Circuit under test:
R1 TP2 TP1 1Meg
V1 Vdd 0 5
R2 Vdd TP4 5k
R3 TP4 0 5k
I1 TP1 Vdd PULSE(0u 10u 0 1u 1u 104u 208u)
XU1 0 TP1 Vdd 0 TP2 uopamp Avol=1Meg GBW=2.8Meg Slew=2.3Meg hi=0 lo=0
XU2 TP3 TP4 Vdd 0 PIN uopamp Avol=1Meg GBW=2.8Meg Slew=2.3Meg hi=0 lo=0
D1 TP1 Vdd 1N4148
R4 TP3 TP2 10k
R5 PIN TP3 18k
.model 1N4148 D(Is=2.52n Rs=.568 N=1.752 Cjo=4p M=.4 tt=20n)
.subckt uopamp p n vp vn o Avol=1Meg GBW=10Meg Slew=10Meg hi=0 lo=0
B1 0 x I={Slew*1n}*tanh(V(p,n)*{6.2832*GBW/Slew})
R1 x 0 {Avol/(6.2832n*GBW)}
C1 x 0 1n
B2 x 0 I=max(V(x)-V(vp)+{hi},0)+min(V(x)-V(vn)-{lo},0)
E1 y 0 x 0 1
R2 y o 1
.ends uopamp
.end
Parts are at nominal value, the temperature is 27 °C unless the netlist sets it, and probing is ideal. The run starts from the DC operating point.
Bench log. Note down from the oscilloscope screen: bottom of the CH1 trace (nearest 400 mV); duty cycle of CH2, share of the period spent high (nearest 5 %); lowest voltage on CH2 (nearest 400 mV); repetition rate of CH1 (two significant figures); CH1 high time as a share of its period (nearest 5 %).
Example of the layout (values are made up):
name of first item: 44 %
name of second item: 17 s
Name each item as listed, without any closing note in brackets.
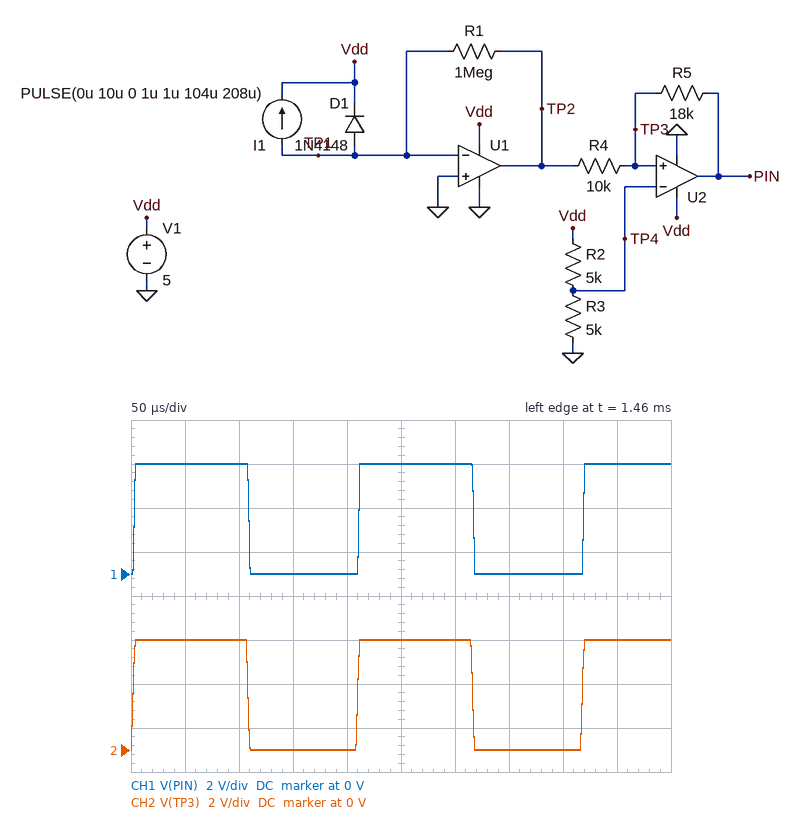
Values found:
bottom of the CH1 trace: 0 V
duty cycle of CH2, share of the period spent high: 50 %
lowest voltage on CH2: 0 V
repetition rate of CH1: 4.8 kHz
CH1 high time as a share of its period: 50 %
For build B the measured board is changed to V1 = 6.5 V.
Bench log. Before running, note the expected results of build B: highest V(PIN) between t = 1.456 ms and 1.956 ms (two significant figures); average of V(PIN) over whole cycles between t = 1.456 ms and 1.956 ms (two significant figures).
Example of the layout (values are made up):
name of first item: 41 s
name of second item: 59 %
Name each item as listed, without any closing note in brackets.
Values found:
highest V(PIN) between t = 1.456 ms and 1.956 ms: 6.5 V
average of V(PIN) over whole cycles between t = 1.456 ms and 1.956 ms: 3.3 V
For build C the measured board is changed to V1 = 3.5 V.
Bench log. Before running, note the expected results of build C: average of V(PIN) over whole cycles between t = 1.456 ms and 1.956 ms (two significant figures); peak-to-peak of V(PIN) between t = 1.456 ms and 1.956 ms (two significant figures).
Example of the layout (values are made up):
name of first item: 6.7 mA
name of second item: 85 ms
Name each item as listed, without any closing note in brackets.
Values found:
average of V(PIN) over whole cycles between t = 1.456 ms and 1.956 ms: 1.8 V
peak-to-peak of V(PIN) between t = 1.456 ms and 1.956 ms: 3.5 V
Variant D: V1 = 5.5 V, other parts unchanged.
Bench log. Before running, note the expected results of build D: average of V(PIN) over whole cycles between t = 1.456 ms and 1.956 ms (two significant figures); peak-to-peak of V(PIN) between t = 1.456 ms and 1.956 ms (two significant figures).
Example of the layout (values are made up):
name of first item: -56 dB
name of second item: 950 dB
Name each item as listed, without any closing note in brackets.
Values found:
average of V(PIN) over whole cycles between t = 1.456 ms and 1.956 ms: 2.8 V
peak-to-peak of V(PIN) between t = 1.456 ms and 1.956 ms: 5.5 V
